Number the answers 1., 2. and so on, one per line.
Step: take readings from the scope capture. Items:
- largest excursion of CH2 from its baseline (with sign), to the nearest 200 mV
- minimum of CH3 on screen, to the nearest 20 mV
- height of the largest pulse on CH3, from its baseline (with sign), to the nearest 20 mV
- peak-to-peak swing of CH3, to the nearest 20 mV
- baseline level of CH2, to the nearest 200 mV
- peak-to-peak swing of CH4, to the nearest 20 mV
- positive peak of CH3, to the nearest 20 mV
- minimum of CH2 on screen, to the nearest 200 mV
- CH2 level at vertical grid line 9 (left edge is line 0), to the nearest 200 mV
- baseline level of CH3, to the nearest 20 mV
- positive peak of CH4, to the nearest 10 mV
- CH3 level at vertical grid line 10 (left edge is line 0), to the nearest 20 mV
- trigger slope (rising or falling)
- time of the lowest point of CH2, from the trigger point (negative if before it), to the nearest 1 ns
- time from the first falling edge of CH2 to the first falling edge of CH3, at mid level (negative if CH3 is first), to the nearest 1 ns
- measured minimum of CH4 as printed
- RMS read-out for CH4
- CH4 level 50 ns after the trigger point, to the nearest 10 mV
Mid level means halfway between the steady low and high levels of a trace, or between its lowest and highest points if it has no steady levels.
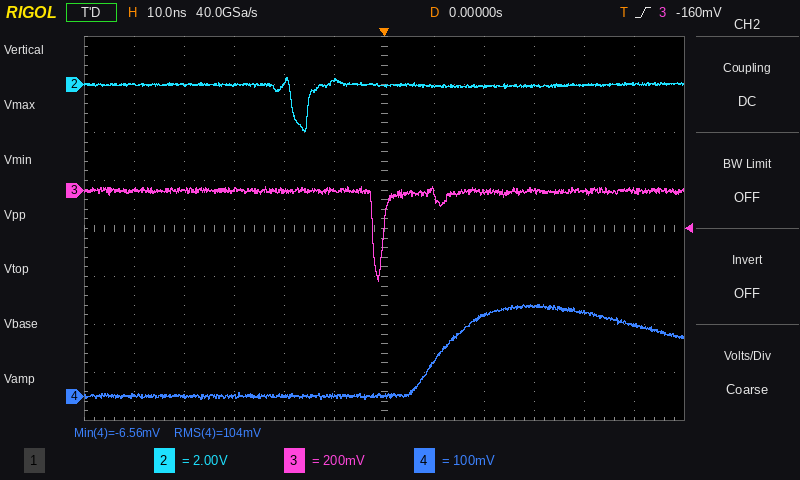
1. -2.0 V
2. -380 mV
3. -380 mV
4. 400 mV
5. 0.0 V
6. 200 mV
7. 20 mV
8. -2.0 V
9. 0.0 V
10. 0 mV
11. 190 mV
12. 0 mV
13. rising
14. -16 ns
15. +16 ns
16. -6.56 mV
17. 104 mV
18. 150 mV
